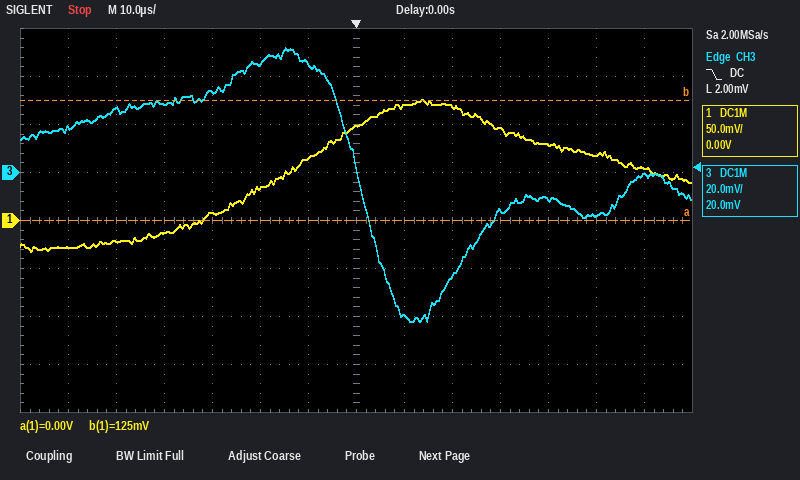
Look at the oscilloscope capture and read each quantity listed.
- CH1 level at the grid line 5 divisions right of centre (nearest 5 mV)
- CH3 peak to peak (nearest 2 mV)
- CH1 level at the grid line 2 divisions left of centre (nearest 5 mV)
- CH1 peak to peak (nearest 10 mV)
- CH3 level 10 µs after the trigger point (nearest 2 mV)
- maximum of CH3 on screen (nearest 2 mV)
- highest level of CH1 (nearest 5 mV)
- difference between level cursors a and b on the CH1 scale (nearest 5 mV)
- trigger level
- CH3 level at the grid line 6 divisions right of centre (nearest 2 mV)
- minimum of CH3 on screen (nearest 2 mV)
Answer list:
70 mV
114 mV
35 mV
160 mV
-60 mV
52 mV
125 mV
125 mV
2.00 mV
0 mV
-62 mV
